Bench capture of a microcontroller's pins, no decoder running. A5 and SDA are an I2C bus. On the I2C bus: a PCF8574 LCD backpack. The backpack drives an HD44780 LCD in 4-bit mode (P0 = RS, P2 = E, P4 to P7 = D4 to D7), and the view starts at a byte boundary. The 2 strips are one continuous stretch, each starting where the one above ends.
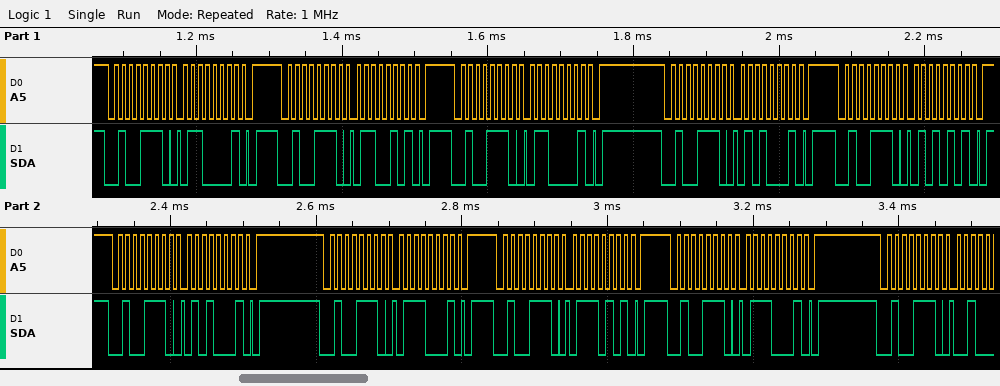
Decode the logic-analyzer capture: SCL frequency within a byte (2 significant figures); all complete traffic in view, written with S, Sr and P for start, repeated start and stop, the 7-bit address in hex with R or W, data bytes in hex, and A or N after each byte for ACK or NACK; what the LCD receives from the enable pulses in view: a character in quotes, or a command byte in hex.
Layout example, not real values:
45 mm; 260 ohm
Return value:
100 kHz; S 27W A 61 A P S 27W A 65 A P S 27W A 61 A P S 27W A 51 A P S 27W A 55 A P S 27W A 51 A P S 27W A 71 A P S 27W A 75 A P S 27W A 71 A P S 27W A; 'e'
